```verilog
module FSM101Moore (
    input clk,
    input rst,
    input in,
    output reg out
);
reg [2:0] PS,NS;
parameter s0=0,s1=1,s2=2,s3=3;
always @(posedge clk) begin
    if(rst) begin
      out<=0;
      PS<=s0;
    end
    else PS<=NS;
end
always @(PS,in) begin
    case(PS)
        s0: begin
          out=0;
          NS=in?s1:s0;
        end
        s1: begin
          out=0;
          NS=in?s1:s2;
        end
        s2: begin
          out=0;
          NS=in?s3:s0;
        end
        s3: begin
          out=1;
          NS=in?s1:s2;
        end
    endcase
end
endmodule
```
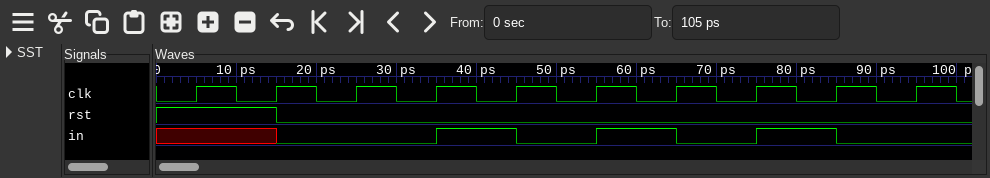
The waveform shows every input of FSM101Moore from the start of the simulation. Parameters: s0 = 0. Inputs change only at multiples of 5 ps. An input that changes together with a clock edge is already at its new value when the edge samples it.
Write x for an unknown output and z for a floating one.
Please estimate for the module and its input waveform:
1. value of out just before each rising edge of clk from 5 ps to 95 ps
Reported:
x 0 0 0 0 0 1 0 1 0
